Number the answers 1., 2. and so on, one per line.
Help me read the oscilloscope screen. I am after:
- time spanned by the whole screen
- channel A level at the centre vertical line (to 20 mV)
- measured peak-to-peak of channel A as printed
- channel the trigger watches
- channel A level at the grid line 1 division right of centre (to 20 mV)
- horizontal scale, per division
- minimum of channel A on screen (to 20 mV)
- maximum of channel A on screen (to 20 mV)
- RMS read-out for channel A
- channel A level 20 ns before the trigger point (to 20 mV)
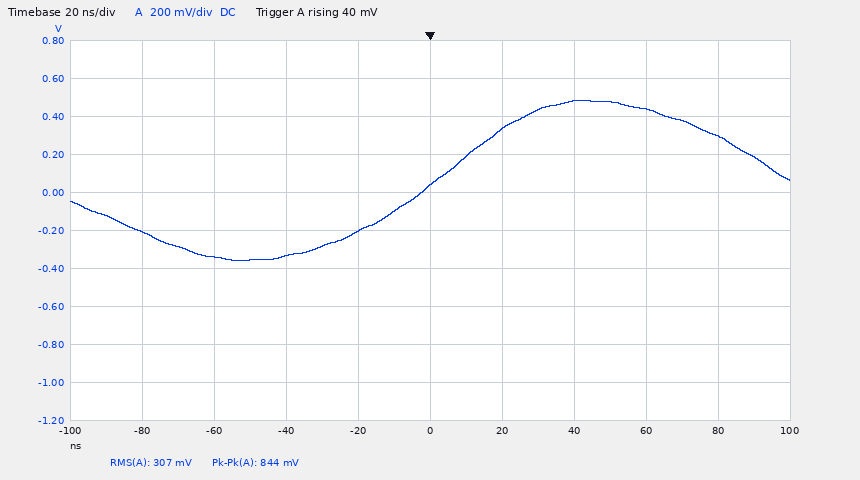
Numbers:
1. 200 ns
2. 40 mV
3. 844 mV
4. channel A
5. 340 mV
6. 20 ns
7. -360 mV
8. 480 mV
9. 307 mV
10. -200 mV
